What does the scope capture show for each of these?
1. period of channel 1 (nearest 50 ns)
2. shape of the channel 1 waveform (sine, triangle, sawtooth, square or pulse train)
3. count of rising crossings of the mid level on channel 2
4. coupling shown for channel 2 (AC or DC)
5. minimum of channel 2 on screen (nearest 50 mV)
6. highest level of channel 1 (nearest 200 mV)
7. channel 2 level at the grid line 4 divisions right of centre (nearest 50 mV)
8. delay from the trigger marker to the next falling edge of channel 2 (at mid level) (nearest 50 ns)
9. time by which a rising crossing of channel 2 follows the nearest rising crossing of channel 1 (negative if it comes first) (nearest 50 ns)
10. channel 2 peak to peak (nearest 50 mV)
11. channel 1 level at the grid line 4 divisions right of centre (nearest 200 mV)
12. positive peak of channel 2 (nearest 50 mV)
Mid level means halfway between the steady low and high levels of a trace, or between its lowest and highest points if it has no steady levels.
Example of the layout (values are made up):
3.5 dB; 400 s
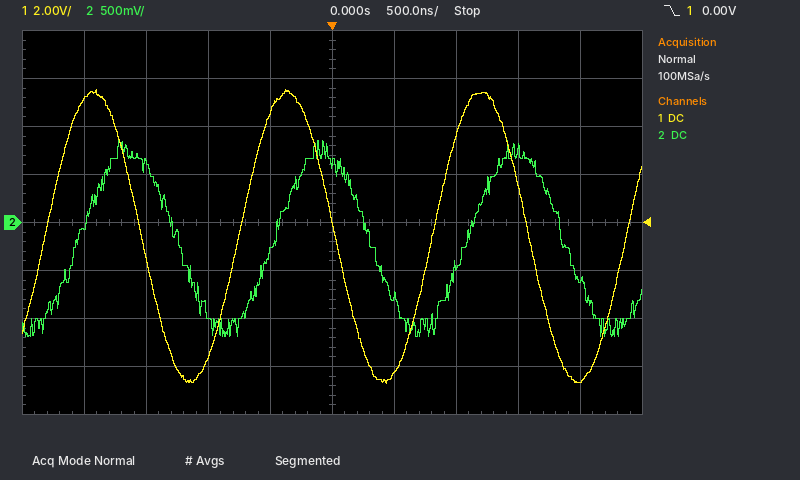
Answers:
1.55 µs; sine; 3; DC; -1.20 V; 5.6 V; -600 mV; 300 ns; +300 ns; 2.05 V; -6.6 V; 850 mV
